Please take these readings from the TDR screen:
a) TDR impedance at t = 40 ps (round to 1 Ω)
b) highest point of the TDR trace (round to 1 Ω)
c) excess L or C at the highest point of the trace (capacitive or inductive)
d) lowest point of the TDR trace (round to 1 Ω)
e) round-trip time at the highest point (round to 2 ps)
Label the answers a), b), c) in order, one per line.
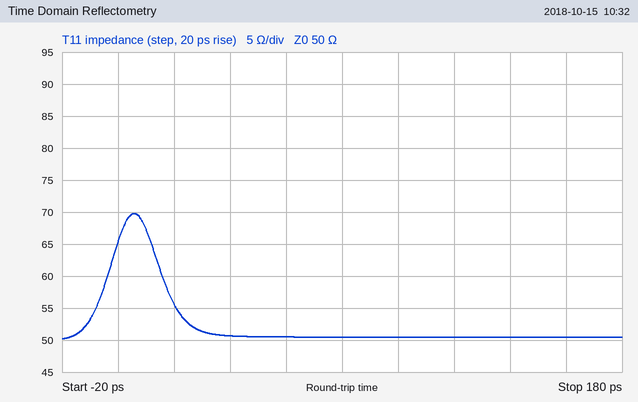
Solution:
a) 51 Ω
b) 70 Ω
c) inductive
d) 50 Ω
e) 6 ps
